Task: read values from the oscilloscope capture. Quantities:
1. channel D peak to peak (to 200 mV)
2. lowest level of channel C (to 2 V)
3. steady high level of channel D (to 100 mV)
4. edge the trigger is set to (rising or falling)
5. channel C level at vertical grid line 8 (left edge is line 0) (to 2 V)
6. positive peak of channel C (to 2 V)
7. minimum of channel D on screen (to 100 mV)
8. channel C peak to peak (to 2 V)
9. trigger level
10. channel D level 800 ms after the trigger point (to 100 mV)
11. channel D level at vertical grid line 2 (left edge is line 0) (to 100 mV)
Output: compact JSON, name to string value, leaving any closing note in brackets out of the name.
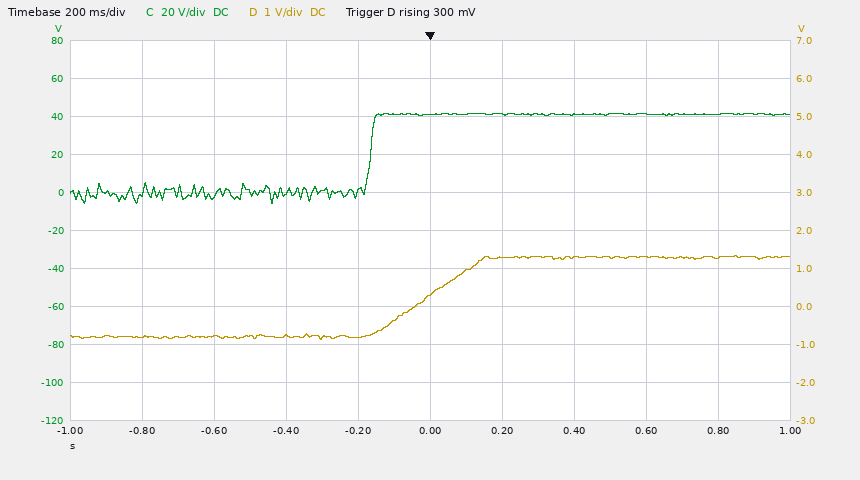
{"channel D peak to peak": "2.2 V", "lowest level of channel C": "-6 V", "steady high level of channel D": "1.3 V", "edge the trigger is set to": "rising", "channel C level at vertical grid line 8 (left edge is line 0)": "42 V", "positive peak of channel C": "42 V", "minimum of channel D on screen": "-900 mV", "channel C peak to peak": "48 V", "trigger level": "300 mV", "channel D level 800 ms after the trigger point": "1.3 V", "channel D level at vertical grid line 2 (left edge is line 0)": "-800 mV"}
